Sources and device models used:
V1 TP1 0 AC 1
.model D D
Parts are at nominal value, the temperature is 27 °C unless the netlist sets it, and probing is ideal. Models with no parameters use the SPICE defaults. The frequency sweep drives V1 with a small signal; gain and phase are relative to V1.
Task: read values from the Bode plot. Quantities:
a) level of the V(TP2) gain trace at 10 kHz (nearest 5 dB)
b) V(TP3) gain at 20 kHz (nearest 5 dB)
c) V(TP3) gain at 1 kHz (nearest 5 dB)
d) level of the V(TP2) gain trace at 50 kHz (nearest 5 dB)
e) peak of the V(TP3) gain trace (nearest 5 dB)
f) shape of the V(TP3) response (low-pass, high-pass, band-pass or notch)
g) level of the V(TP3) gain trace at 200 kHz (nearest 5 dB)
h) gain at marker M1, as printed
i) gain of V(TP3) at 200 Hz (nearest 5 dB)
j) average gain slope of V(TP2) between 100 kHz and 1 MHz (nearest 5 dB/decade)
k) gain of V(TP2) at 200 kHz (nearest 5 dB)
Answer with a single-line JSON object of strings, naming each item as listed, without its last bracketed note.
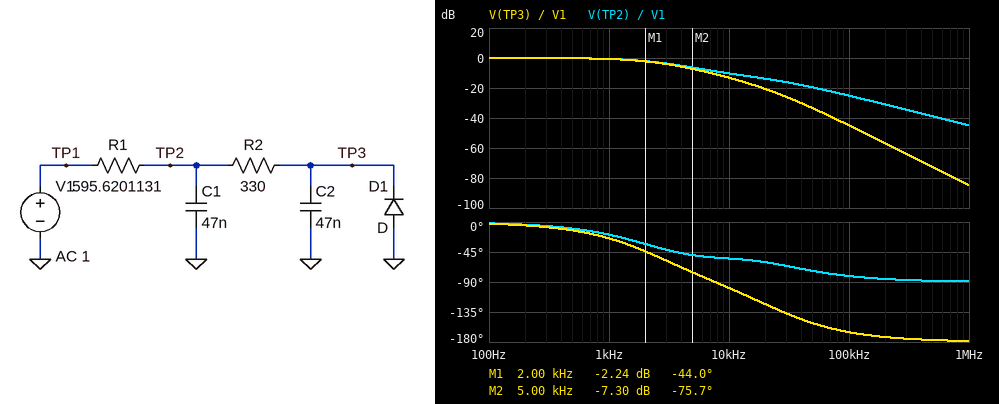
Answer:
{"level of the V(TP2) gain trace at 10 kHz": "-10 dB", "V(TP3) gain at 20 kHz": "-20 dB", "V(TP3) gain at 1 kHz": "0 dB", "level of the V(TP2) gain trace at 50 kHz": "-20 dB", "peak of the V(TP3) gain trace": "0 dB", "shape of the V(TP3) response": "low-pass", "level of the V(TP3) gain trace at 200 kHz": "-55 dB", "gain at marker M1, as printed": "-2.24 dB", "gain of V(TP3) at 200 Hz": "0 dB", "average gain slope of V(TP2) between 100 kHz and 1 MHz": "-20 dB/decade", "gain of V(TP2) at 200 kHz": "-30 dB"}
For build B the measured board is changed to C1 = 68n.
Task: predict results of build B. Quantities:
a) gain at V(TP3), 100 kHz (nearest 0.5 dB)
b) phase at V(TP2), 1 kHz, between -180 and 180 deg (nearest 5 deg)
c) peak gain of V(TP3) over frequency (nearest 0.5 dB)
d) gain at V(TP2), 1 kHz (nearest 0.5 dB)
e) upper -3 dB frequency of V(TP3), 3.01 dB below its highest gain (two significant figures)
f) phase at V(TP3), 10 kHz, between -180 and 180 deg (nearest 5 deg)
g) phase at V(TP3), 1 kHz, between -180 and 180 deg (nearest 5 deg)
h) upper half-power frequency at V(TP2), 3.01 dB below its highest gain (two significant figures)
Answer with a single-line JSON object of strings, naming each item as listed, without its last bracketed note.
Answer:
{"gain at V(TP3), 100 kHz": "-48.0 dB", "phase at V(TP2), 1 kHz, between -180 and 180 deg": "-25 deg", "peak gain of V(TP3) over frequency": "0 dB", "gain at V(TP2), 1 kHz": "-1.0 dB", "upper -3 dB frequency of V(TP3), 3.01 dB below its highest gain": "2.1 kHz", "phase at V(TP3), 10 kHz, between -180 and 180 deg": "-105 deg", "phase at V(TP3), 1 kHz, between -180 and 180 deg": "-30 deg", "upper half-power frequency at V(TP2), 3.01 dB below its highest gain": "2.2 kHz"}
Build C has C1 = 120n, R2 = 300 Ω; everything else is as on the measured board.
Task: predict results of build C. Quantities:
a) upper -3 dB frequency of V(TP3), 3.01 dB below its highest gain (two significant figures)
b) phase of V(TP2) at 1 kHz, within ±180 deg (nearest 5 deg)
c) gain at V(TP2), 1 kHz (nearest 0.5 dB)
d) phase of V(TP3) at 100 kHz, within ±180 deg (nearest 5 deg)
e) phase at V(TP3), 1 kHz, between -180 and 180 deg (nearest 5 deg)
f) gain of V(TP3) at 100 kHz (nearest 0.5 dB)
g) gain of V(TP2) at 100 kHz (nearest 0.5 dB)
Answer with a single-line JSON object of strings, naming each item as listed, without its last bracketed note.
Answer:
{"upper -3 dB frequency of V(TP3), 3.01 dB below its highest gain": "1.5 kHz", "phase of V(TP2) at 1 kHz, within ±180 deg": "-30 deg", "gain at V(TP2), 1 kHz": "-1.5 dB", "phase of V(TP3) at 100 kHz, within ±180 deg": "-170 deg", "phase at V(TP3), 1 kHz, between -180 and 180 deg": "-35 deg", "gain of V(TP3) at 100 kHz": "-52.0 dB", "gain of V(TP2) at 100 kHz": "-33.0 dB"}
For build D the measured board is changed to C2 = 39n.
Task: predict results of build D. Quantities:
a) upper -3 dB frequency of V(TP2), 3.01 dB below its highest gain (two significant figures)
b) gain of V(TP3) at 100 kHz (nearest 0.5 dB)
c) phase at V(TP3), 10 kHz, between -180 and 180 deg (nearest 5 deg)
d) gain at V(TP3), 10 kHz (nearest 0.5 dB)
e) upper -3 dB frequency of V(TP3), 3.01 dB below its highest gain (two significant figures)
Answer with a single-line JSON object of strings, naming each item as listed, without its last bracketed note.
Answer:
{"upper -3 dB frequency of V(TP2), 3.01 dB below its highest gain": "2.9 kHz", "gain of V(TP3) at 100 kHz": "-43.5 dB", "phase at V(TP3), 10 kHz, between -180 and 180 deg": "-95 deg", "gain at V(TP3), 10 kHz": "-12.0 dB", "upper -3 dB frequency of V(TP3), 3.01 dB below its highest gain": "2.7 kHz"}
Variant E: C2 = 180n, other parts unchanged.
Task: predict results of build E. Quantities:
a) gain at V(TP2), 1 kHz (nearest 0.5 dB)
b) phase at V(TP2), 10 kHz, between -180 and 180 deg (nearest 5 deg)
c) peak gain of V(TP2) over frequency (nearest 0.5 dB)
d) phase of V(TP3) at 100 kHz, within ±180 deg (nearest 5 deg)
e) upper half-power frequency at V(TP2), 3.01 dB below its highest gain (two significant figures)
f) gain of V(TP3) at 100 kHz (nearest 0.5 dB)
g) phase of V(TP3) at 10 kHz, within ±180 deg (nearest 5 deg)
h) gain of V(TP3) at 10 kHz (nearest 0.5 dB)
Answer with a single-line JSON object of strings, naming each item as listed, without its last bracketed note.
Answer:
{"gain at V(TP2), 1 kHz": "-3.0 dB", "phase at V(TP2), 10 kHz, between -180 and 180 deg": "-40 deg", "peak gain of V(TP2) over frequency": "0 dB", "phase of V(TP3) at 100 kHz, within ±180 deg": "-170 deg", "upper half-power frequency at V(TP2), 3.01 dB below its highest gain": "960 Hz", "gain of V(TP3) at 100 kHz": "-56.5 dB", "phase of V(TP3) at 10 kHz, within ±180 deg": "-115 deg", "gain of V(TP3) at 10 kHz": "-22.5 dB"}
